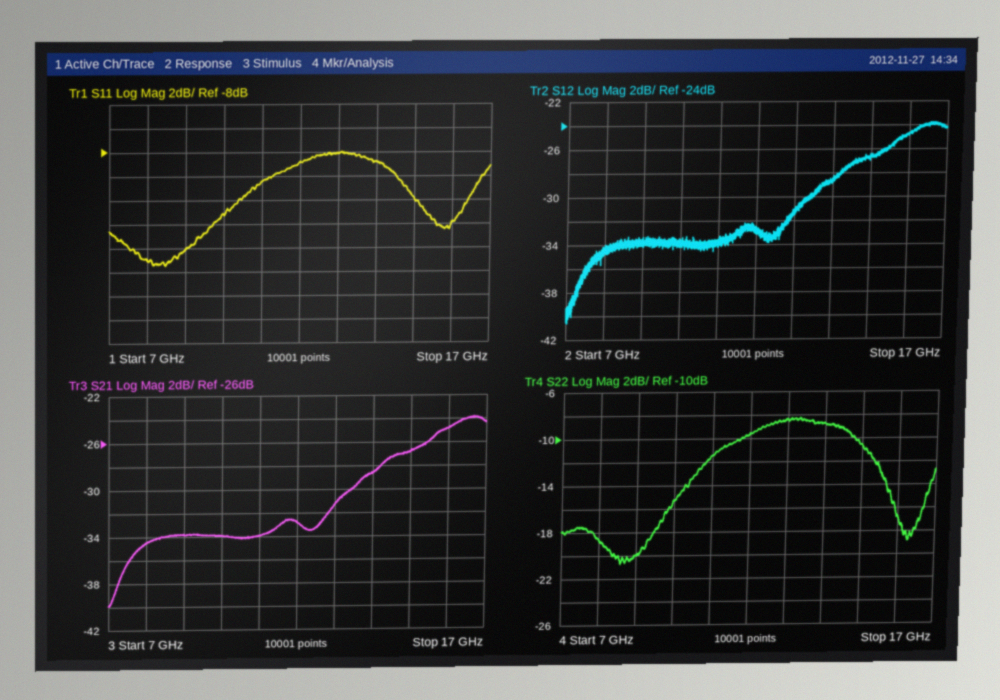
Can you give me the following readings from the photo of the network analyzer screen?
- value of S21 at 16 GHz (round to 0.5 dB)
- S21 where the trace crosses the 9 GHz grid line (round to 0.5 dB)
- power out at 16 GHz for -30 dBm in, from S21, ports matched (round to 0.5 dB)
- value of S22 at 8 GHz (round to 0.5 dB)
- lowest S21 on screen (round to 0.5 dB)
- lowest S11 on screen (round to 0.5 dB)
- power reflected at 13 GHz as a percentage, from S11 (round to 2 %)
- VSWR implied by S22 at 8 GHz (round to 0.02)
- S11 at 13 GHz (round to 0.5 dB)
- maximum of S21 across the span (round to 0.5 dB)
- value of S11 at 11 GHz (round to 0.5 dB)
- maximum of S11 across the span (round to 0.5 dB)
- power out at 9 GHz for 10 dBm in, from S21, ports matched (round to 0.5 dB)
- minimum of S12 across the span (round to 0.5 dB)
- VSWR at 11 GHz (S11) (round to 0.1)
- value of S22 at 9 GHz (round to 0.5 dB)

-25.0 dB
-34.0 dB
-55.0 dBm
-18.5 dB
-40.0 dB
-17.5 dB
16 %
1.26
-8.0 dB
-24.0 dB
-10.5 dB
-8.0 dB
-24.0 dBm
-40.5 dB
1.9
-20.0 dB
